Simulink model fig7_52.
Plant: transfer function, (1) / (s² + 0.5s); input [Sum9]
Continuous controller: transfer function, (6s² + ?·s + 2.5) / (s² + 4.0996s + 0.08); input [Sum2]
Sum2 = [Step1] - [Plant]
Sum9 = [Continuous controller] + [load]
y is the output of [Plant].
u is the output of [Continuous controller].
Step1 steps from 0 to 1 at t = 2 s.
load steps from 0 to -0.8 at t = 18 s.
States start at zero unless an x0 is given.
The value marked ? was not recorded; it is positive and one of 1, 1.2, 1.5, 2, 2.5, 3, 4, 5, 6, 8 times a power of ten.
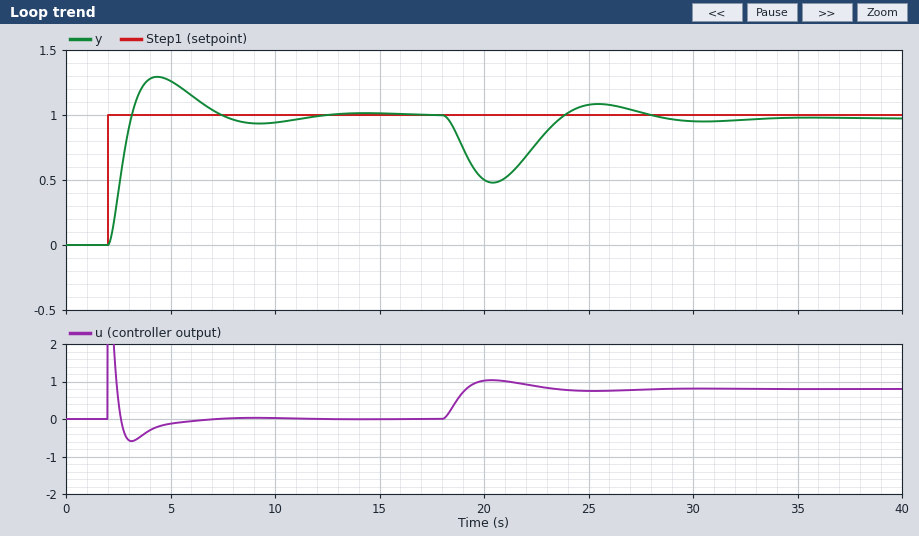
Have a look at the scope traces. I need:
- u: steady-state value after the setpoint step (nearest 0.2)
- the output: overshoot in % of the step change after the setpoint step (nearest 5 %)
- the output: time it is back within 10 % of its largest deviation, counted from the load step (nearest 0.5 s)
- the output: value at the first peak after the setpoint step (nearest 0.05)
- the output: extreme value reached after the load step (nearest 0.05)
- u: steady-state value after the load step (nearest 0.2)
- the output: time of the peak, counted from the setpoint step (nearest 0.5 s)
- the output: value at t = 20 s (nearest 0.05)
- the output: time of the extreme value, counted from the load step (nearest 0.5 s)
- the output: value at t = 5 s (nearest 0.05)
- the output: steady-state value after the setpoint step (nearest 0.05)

0.0
30 %
9.5 s
1.30
0.50
0.8
2.5 s
0.50
2.5 s
1.25
1.00
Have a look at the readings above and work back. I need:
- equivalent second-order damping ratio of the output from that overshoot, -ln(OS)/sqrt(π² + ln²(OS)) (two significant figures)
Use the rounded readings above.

0.36
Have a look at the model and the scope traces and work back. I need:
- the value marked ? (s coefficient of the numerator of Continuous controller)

5
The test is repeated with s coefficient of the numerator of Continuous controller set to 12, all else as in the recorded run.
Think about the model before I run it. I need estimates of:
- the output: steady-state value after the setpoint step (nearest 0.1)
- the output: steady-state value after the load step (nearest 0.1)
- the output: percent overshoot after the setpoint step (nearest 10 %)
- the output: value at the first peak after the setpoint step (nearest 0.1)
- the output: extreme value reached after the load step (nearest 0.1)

1.0
1.0
50 %
1.5
0.7
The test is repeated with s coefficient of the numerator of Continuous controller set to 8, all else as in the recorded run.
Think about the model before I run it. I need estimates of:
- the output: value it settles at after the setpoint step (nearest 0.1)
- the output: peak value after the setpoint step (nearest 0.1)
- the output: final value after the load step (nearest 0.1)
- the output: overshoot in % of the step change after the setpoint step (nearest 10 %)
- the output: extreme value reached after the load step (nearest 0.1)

1.0
1.4
1.0
40 %
0.6
